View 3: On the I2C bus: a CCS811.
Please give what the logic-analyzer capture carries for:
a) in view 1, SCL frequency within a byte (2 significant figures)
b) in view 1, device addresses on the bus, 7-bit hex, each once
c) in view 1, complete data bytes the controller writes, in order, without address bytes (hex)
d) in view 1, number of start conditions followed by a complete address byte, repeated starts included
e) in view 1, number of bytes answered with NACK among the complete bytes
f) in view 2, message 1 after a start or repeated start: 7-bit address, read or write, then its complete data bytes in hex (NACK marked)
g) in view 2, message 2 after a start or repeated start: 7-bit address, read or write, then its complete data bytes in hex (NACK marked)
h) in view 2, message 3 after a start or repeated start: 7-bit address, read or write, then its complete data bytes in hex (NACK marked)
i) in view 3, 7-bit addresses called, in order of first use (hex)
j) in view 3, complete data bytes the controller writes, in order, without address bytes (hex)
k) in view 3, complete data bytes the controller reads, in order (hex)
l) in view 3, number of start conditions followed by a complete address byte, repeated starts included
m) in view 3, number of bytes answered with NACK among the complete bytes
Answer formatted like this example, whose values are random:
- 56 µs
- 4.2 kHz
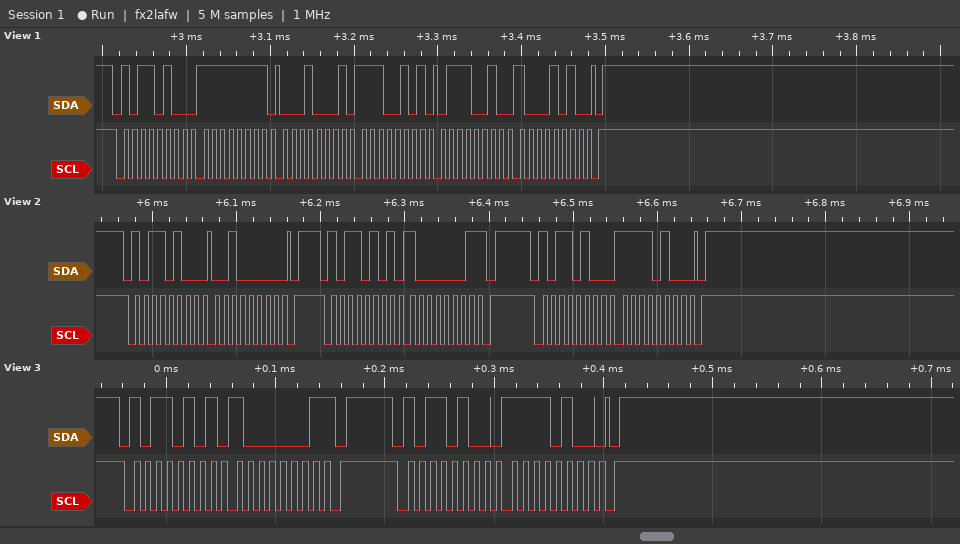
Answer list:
- 100 kHz
- 0x5A
- FF 11 E5 72 8A
- 1
- 0
- 0x5A write: 20
- 0x5A read: 81 NACK
- 0x5A write: F4
- 0x5A
- F4
- 81
- 2
- 1
